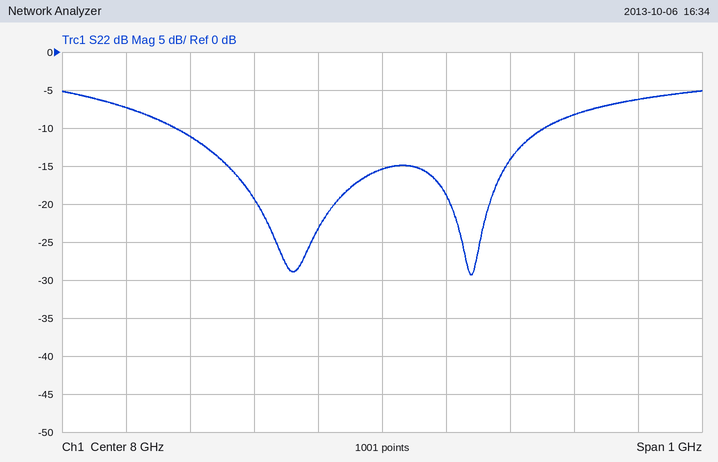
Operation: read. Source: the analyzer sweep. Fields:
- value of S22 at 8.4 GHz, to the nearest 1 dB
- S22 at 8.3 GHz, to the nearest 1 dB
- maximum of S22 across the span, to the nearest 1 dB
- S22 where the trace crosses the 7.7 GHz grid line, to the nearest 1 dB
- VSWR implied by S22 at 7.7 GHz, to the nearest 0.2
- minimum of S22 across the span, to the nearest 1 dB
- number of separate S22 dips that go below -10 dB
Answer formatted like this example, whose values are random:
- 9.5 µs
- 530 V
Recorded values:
- -6 dB
- -8 dB
- -5 dB
- -11 dB
- 1.8
- -29 dB
- 2
